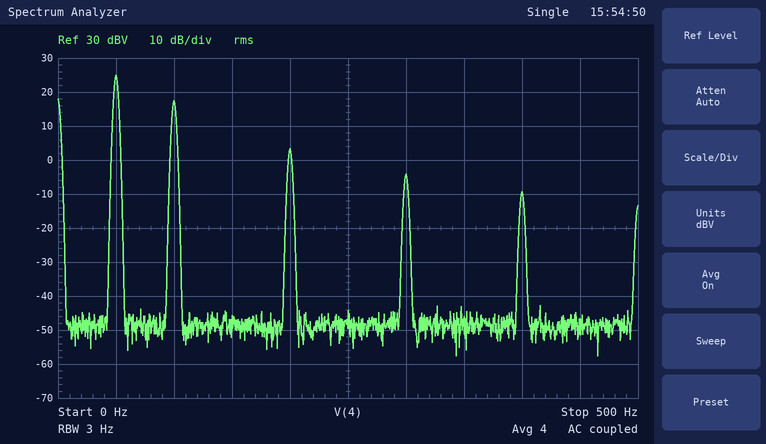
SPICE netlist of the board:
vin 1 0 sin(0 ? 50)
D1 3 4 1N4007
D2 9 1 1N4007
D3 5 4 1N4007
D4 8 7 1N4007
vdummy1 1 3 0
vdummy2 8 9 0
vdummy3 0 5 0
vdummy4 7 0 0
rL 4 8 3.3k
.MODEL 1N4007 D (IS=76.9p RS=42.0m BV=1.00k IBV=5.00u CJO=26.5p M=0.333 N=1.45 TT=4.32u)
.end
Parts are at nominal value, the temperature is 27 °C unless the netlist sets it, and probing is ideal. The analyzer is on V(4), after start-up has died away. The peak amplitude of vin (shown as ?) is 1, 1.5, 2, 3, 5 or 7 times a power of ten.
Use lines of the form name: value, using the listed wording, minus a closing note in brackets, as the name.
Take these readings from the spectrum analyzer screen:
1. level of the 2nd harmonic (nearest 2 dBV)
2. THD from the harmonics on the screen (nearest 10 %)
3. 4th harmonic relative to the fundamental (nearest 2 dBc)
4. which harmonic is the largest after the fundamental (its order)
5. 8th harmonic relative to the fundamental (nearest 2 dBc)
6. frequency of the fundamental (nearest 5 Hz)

level of the 2nd harmonic: 18 dBV
THD from the harmonics on the screen: 40 %
4th harmonic relative to the fundamental: -22 dBc
which harmonic is the largest after the fundamental: 2
8th harmonic relative to the fundamental: -34 dBc
frequency of the fundamental: 50 Hz
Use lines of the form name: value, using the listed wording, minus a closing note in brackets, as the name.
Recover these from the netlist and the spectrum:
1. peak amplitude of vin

peak amplitude of vin: 50 V
